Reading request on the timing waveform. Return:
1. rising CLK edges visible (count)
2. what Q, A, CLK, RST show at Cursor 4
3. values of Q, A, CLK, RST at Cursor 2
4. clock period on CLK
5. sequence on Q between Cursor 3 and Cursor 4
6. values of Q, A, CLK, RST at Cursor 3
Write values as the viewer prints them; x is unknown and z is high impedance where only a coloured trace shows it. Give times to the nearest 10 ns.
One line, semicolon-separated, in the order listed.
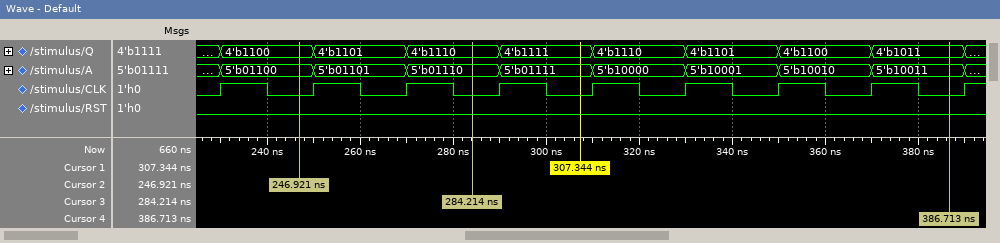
9; Q=4'b1011, A=5'b10011, CLK=0, RST=0; Q=4'b1100, A=5'b01100, CLK=0, RST=0; 20 ns; 4'b1110, 4'b1111, 4'b1110, 4'b1101, 4'b1100, 4'b1011; Q=4'b1110, A=5'b01110, CLK=0, RST=0
